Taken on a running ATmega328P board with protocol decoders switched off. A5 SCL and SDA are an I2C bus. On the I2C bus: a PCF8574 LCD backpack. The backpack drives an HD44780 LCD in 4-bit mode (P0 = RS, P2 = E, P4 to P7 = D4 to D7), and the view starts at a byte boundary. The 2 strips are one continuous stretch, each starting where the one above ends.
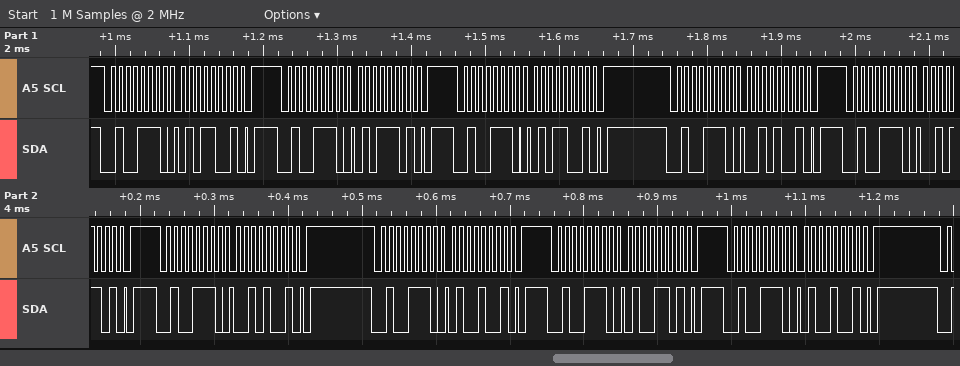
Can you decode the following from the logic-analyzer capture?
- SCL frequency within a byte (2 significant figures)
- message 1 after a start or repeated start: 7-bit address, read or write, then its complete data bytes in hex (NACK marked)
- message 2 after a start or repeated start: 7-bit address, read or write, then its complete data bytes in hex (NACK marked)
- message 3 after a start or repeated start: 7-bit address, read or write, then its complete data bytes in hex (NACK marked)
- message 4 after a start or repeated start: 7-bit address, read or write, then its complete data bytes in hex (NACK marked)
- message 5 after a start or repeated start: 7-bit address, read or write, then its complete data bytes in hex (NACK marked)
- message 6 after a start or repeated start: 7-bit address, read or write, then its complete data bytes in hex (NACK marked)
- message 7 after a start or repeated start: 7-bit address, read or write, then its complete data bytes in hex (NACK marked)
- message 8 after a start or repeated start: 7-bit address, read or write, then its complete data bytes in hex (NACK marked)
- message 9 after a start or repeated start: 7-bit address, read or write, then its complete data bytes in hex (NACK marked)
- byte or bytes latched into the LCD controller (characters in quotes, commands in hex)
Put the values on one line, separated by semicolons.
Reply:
100 kHz; 0x27 write: 59; 0x27 write: 5D; 0x27 write: 59; 0x27 write: 29; 0x27 write: 2D; 0x27 write: 29; 0x27 write: 49; 0x27 write: 4D; 0x27 write: 49; 'R'
